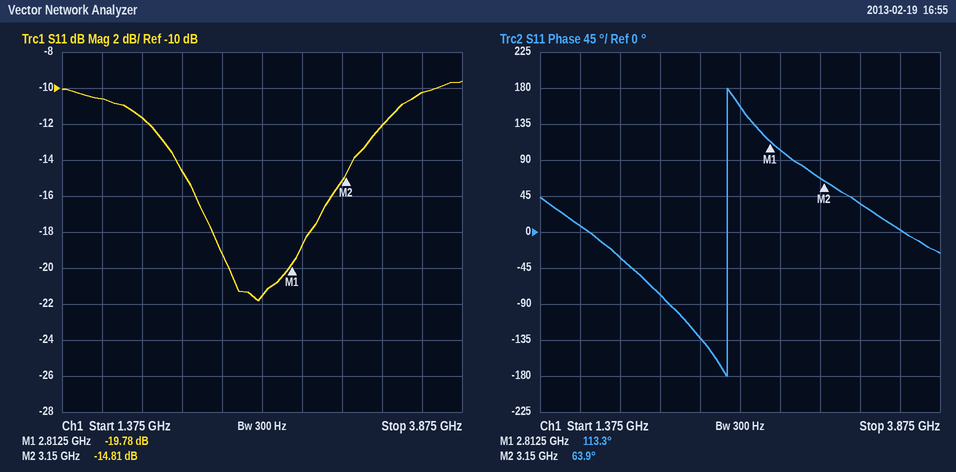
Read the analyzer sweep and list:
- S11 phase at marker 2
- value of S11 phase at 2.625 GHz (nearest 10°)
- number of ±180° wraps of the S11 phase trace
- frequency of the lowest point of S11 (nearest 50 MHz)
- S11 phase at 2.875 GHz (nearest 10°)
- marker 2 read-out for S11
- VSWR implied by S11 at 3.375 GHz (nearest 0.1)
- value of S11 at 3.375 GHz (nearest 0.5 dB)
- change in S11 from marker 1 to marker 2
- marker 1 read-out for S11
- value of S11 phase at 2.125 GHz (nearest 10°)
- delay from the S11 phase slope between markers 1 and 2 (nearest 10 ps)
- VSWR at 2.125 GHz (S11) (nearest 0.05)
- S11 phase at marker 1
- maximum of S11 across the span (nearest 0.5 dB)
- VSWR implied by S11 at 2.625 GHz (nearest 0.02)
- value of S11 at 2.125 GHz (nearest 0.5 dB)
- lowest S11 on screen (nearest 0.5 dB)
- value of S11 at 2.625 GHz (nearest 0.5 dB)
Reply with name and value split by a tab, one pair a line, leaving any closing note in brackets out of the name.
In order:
S11 phase at marker 2	63.9°
value of S11 phase at 2.625 GHz	160°
number of ±180° wraps of the S11 phase trace	1
frequency of the lowest point of S11	2.60 GHz
S11 phase at 2.875 GHz	100°
marker 2 read-out for S11	-14.81 dB
VSWR implied by S11 at 3.375 GHz	1.7
value of S11 at 3.375 GHz	-12.0 dB
change in S11 from marker 1 to marker 2	4.97 dB
marker 1 read-out for S11	-19.78 dB
value of S11 phase at 2.125 GHz	-80°
delay from the S11 phase slope between markers 1 and 2	410 ps
VSWR at 2.125 GHz (S11)	1.45
S11 phase at marker 1	113.3°
maximum of S11 across the span	-9.5 dB
VSWR implied by S11 at 2.625 GHz	1.18
value of S11 at 2.125 GHz	-14.5 dB
lowest S11 on screen	-22.0 dB
value of S11 at 2.625 GHz	-21.5 dB
